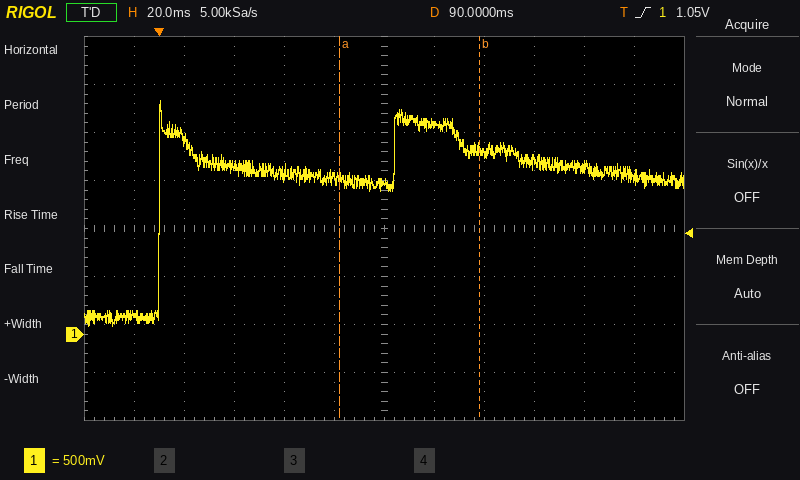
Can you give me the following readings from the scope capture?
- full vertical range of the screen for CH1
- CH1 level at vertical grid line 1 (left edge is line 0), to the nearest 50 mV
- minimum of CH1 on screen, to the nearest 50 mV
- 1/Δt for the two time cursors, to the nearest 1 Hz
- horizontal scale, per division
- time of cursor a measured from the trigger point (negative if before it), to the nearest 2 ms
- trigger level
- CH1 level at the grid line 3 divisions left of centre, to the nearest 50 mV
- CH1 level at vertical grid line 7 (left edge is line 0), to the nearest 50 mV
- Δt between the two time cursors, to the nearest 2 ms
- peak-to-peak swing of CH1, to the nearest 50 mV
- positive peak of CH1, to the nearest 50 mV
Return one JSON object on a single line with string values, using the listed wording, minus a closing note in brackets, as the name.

{"full vertical range of the screen for CH1": "4 V", "CH1 level at vertical grid line 1 (left edge is line 0), to the nearest 50 mV": "200 mV", "minimum of CH1 on screen, to the nearest 50 mV": "100 mV", "1/Δt for the two time cursors, to the nearest 1 Hz": "18 Hz", "horizontal scale, per division": "20 ms", "time of cursor a measured from the trigger point (negative if before it), to the nearest 2 ms": "+72 ms", "trigger level": "1.05 V", "CH1 level at the grid line 3 divisions left of centre, to the nearest 50 mV": "1.75 V", "CH1 level at vertical grid line 7 (left edge is line 0), to the nearest 50 mV": "2.20 V", "Δt between the two time cursors, to the nearest 2 ms": "56 ms", "peak-to-peak swing of CH1, to the nearest 50 mV": "2.35 V", "positive peak of CH1, to the nearest 50 mV": "2.45 V"}
